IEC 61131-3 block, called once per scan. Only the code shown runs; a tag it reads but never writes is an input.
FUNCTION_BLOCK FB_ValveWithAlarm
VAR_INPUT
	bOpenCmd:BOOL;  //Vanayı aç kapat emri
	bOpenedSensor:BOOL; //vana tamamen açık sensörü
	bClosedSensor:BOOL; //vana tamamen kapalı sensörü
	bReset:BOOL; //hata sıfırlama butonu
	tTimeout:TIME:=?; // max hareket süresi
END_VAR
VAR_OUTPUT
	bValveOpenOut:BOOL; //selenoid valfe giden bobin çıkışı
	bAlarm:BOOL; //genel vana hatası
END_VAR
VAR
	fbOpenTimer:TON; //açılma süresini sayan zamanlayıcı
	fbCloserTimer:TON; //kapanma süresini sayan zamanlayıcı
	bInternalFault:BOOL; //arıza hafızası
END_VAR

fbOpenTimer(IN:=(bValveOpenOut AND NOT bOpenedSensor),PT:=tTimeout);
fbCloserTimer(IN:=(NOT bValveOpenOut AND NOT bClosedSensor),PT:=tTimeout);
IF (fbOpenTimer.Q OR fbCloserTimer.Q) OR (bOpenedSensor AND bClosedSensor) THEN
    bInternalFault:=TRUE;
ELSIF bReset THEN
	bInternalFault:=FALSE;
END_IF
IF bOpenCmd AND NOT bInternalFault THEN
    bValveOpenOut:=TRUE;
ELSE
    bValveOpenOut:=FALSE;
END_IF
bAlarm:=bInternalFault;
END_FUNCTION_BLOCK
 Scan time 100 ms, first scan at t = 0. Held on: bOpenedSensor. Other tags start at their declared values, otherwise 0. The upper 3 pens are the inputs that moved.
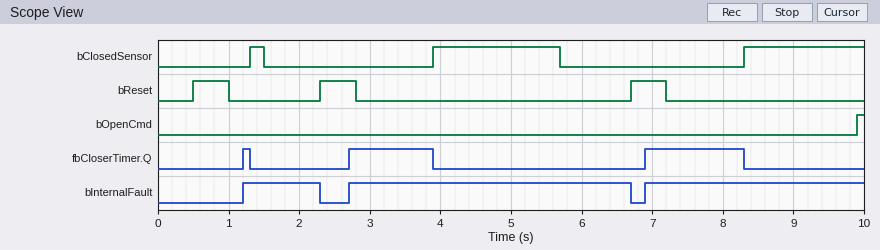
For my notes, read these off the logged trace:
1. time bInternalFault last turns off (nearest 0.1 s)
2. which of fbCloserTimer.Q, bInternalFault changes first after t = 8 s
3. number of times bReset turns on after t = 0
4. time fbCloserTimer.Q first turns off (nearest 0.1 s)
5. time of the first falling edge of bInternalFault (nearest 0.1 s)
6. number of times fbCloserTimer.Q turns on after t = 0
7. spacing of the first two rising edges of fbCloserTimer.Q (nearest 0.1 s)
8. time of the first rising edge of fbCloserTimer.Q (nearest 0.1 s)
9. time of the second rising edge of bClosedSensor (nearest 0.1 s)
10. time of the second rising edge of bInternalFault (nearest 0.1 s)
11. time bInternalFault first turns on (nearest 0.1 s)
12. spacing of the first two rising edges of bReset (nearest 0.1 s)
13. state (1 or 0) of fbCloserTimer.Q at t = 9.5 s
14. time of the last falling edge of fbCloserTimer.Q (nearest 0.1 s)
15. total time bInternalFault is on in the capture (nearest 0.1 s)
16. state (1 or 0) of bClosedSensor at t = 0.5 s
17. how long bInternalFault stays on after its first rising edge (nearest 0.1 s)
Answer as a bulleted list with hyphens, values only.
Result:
- 6.7 s
- fbCloserTimer.Q
- 3
- 1.3 s
- 2.3 s
- 3
- 1.5 s
- 1.2 s
- 3.9 s
- 2.7 s
- 1.2 s
- 1.8 s
- 0
- 8.3 s
- 8.2 s
- 0
- 1.1 s
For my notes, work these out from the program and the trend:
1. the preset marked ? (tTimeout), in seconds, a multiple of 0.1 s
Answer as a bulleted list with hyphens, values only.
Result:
- 1.2 s
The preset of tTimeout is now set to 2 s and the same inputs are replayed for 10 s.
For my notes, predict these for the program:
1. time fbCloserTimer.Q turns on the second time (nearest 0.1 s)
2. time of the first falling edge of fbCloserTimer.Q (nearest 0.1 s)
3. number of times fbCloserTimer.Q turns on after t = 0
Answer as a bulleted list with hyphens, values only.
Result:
- 7.7 s
- 3.9 s
- 2
